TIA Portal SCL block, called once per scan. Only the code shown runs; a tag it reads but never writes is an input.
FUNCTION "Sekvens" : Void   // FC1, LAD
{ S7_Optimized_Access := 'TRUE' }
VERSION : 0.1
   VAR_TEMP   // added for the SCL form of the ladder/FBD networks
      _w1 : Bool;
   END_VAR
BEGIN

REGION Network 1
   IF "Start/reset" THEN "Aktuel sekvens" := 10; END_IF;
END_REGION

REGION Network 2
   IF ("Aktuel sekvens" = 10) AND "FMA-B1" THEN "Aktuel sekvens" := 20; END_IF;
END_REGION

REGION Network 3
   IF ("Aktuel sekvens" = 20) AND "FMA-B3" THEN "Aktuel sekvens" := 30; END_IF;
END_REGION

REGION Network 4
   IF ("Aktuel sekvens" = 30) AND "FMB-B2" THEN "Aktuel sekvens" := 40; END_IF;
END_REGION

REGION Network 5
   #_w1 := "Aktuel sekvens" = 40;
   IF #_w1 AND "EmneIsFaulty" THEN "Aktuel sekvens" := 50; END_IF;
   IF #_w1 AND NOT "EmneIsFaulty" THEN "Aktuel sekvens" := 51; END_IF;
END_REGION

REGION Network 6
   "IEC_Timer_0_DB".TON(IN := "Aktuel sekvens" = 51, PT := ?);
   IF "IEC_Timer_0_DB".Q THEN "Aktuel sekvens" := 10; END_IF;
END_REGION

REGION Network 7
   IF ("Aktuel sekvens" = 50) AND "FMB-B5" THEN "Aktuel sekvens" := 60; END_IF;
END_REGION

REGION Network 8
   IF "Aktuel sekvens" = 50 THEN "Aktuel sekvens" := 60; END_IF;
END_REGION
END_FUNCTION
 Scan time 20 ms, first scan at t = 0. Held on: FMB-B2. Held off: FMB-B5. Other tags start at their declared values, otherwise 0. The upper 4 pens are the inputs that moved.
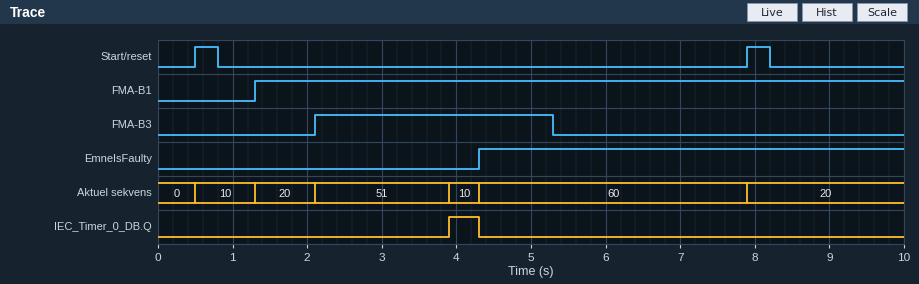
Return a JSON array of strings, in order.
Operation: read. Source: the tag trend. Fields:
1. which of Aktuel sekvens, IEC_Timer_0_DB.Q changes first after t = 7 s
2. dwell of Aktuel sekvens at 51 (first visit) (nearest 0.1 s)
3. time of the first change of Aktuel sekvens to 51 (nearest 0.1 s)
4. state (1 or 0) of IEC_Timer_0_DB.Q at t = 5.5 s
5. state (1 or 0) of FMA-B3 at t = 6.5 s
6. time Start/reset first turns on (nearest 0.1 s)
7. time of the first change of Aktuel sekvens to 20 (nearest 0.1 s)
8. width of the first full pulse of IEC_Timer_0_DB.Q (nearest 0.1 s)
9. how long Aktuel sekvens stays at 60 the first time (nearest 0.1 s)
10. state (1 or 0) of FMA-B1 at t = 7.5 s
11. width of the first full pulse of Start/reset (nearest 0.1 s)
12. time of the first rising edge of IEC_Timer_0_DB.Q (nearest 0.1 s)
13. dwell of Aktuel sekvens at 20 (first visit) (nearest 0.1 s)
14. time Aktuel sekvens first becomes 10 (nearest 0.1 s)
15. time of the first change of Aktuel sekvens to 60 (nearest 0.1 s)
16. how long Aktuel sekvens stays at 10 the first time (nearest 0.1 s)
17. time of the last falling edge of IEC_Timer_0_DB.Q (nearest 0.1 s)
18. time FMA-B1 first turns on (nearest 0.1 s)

["Aktuel sekvens", "1.8 s", "2.1 s", "0", "0", "0.5 s", "1.3 s", "0.4 s", "3.6 s", "1", "0.3 s", "3.9 s", "0.8 s", "0.5 s", "4.3 s", "0.8 s", "4.3 s", "1.3 s"]
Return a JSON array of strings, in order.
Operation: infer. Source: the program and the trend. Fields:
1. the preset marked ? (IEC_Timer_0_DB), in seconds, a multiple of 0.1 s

["1.8 s"]
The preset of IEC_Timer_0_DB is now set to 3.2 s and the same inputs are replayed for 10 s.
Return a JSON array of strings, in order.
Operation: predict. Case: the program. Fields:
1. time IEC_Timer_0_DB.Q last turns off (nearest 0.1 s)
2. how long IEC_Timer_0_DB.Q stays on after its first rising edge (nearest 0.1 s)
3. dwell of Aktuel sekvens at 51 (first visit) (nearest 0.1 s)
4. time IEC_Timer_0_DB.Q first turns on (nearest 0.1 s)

["5.3 s", "0.0 s", "3.2 s", "5.3 s"]
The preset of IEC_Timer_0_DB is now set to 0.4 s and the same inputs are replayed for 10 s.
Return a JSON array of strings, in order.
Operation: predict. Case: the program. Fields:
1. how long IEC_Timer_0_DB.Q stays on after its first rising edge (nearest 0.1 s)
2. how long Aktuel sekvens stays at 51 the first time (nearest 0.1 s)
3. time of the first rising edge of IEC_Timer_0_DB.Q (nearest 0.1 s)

["1.8 s", "0.4 s", "2.5 s"]
